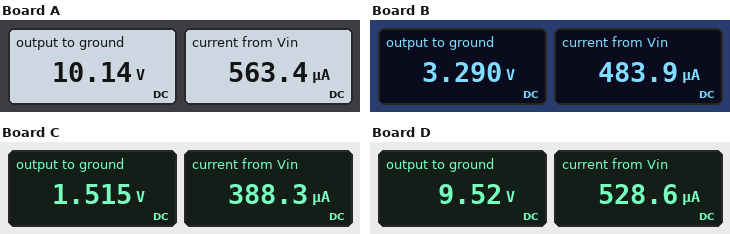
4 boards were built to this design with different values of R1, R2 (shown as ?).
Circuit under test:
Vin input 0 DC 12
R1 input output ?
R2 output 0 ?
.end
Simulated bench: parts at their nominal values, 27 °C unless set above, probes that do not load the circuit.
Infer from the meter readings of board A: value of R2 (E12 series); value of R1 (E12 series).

18 kΩ
3.3 kΩ
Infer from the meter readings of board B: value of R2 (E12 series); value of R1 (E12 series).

6.8 kΩ
18 kΩ
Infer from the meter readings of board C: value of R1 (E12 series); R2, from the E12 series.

27 kΩ
3.9 kΩ
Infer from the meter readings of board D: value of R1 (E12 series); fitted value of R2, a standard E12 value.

4.7 kΩ
18 kΩ
